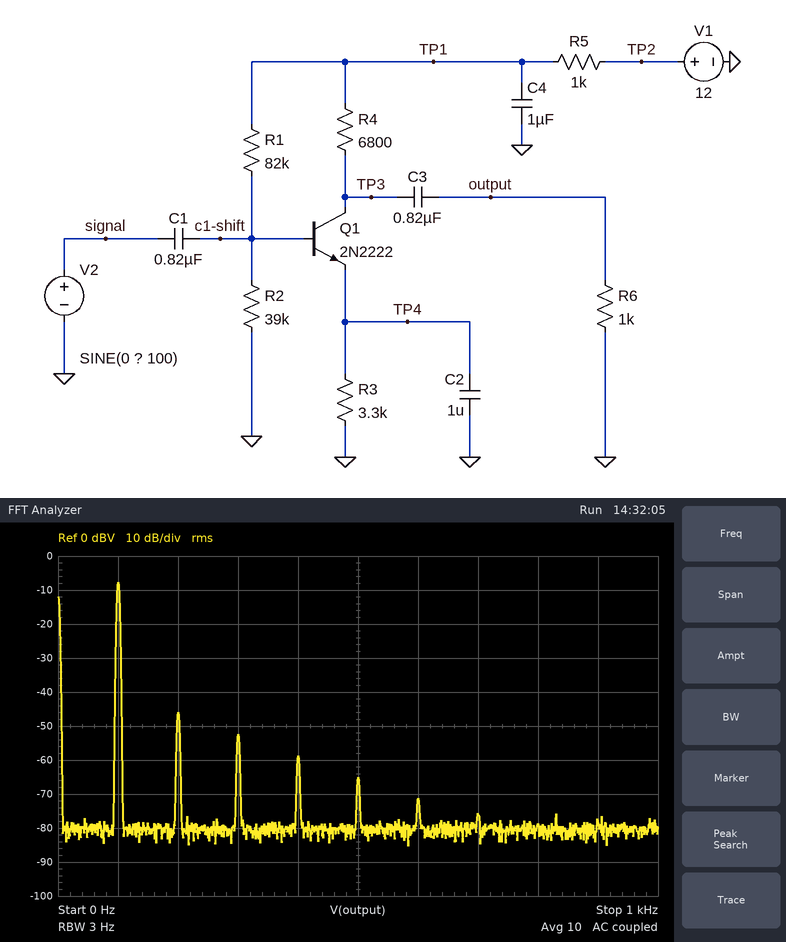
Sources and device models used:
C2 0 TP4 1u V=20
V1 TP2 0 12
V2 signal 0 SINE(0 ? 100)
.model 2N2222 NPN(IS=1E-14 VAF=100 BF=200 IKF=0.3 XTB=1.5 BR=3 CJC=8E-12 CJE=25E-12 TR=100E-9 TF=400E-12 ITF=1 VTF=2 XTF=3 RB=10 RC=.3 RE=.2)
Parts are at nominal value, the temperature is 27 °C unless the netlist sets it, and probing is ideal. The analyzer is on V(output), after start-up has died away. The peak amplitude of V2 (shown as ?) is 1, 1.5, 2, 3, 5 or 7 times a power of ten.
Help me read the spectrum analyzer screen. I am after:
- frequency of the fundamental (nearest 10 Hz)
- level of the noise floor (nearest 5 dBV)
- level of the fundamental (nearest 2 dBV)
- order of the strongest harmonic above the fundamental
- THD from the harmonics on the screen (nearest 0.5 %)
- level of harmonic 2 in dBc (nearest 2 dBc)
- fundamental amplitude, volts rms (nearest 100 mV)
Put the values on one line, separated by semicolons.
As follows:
100 Hz; -80 dBV; -8 dBV; 2; 1.5 %; -38 dBc; 400 mV
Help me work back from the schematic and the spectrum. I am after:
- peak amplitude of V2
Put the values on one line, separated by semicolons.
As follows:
1 V
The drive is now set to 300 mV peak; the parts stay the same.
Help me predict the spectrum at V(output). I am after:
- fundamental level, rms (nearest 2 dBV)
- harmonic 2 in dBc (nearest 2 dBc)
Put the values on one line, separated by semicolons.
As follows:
-18 dBV; -52 dBc
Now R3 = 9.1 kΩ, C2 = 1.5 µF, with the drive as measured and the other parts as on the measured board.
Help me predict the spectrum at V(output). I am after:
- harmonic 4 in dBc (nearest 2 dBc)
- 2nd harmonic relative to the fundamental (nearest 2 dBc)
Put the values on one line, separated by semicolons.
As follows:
-16 dBc; -6 dBc
